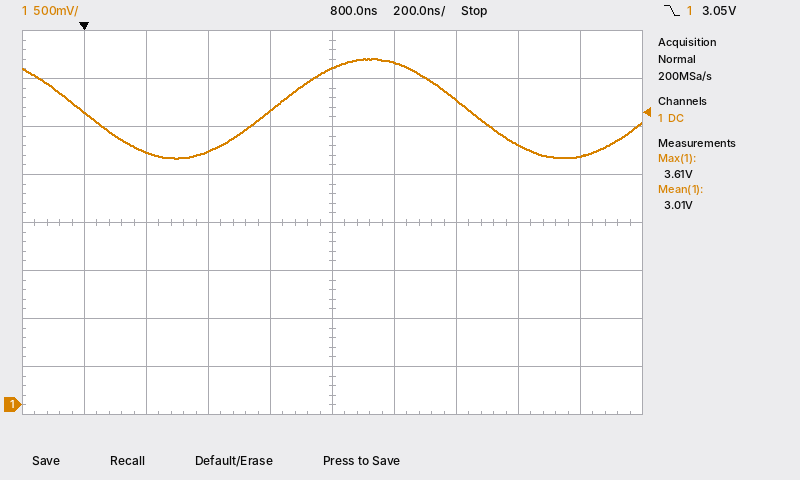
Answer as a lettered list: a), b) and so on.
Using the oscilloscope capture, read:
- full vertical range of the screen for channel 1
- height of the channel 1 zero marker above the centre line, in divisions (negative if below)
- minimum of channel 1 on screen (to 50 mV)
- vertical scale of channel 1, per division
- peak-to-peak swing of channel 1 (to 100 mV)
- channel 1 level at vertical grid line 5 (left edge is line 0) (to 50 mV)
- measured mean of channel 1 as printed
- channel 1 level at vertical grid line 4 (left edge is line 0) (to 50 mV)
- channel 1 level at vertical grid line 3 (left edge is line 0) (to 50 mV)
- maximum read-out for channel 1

a) 4 V
b) -3.8 div
c) 2.55 V
d) 500 mV
e) 1.00 V
f) 3.50 V
g) 3.01 V
h) 3.05 V
i) 2.65 V
j) 3.61 V
